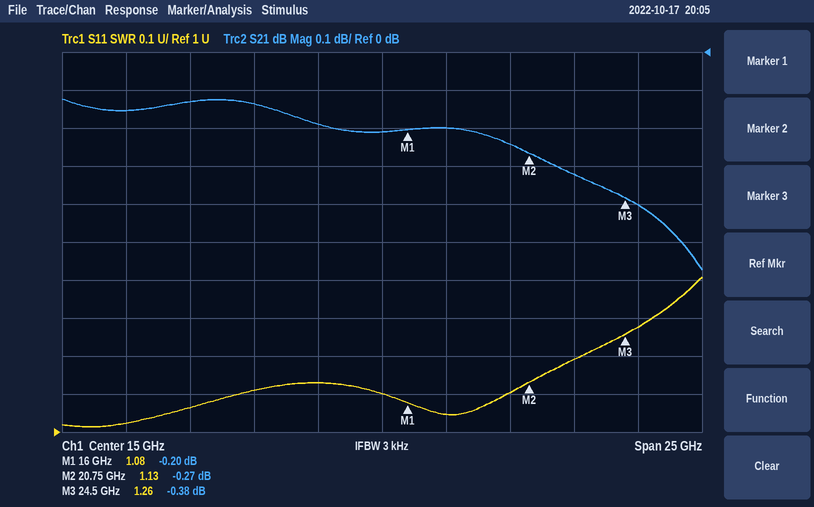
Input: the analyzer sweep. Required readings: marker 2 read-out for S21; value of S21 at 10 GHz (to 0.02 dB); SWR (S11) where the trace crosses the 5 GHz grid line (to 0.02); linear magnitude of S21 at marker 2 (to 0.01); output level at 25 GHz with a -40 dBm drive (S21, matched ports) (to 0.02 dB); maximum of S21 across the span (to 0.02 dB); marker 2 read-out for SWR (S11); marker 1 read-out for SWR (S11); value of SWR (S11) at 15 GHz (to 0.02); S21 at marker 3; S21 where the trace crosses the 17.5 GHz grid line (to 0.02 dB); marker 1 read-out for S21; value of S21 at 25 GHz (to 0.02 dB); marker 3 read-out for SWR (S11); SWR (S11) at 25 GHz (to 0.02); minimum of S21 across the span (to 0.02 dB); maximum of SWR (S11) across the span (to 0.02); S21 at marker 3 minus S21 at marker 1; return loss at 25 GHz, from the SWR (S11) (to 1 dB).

-0.27 dB
-0.14 dB
1.02
0.97
-40.40 dBm
-0.12 dB
1.13
1.08
1.10
-0.38 dB
-0.20 dB
-0.20 dB
-0.40 dB
1.26
1.28
-0.58 dB
1.40
-0.18 dB
18 dB
